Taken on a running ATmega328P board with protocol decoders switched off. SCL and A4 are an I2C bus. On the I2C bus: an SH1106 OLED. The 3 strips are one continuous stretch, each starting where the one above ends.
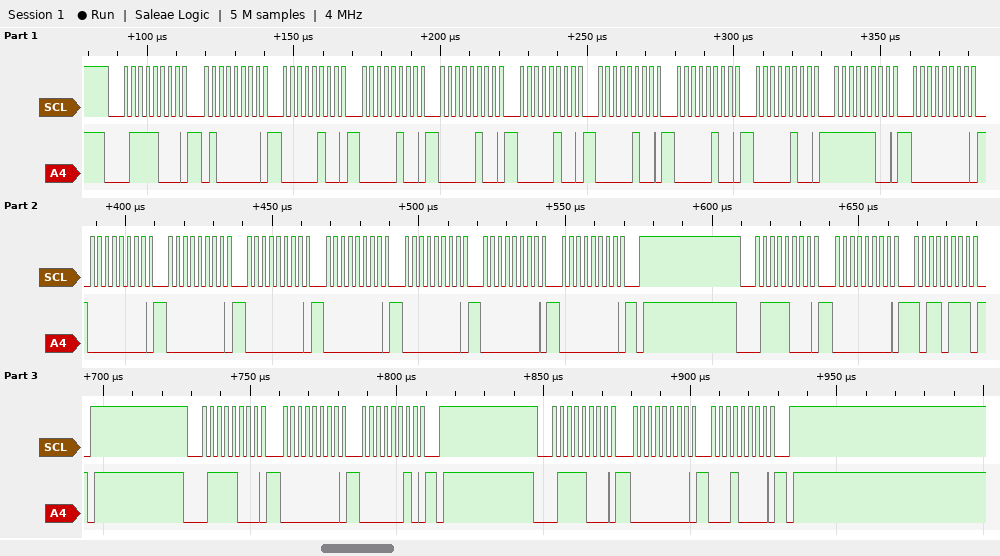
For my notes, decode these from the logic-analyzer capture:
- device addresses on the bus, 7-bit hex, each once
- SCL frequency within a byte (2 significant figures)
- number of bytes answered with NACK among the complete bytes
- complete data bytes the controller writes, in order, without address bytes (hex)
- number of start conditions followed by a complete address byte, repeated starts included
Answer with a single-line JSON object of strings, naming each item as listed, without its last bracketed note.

{"device addresses on the bus, 7-bit hex, each once": "0x3C", "SCL frequency within a byte": "400 kHz", "number of bytes answered with NACK among the complete bytes": "0", "complete data bytes the controller writes, in order, without address bytes": "40 04 04 04 04 04 04 04 FC 00 00 00 00 00 00 00 00 00 B7 00 02 00 10", "number of start conditions followed by a complete address byte, repeated starts included": "4"}
